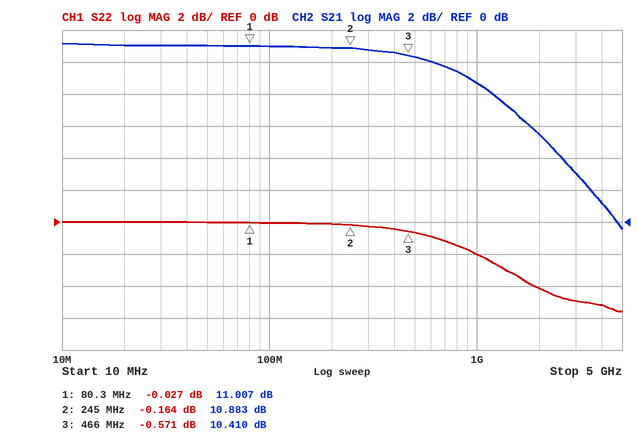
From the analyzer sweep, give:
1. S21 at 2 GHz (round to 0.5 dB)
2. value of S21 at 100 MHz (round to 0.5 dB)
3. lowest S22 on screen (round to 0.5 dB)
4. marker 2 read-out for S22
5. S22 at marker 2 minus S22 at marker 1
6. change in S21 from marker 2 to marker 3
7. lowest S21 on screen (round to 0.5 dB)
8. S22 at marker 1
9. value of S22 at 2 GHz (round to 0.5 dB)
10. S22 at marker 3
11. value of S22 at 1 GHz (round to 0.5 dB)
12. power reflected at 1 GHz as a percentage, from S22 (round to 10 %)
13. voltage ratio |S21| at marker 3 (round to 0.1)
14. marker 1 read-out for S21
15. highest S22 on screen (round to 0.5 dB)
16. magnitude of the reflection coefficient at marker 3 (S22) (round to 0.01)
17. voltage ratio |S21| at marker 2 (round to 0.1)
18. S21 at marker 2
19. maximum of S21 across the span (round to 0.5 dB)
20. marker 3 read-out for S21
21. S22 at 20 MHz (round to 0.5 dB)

5.5 dB
11.0 dB
-5.5 dB
-0.164 dB
-0.137 dB
-0.473 dB
-0.5 dB
-0.027 dB
-4.0 dB
-0.571 dB
-2.0 dB
60 %
3.3
11.007 dB
0.0 dB
0.94
3.5
10.883 dB
11.0 dB
10.410 dB
0.0 dB
